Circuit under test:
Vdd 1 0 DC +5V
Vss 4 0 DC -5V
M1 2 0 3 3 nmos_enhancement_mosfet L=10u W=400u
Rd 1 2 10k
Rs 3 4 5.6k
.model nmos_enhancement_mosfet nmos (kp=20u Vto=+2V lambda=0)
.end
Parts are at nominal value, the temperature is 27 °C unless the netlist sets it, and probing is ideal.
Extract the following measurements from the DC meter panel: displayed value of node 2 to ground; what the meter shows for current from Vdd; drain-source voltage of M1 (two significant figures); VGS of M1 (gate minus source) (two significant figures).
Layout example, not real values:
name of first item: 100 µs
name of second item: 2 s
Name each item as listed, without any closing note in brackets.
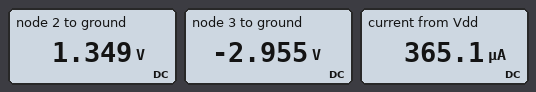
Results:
displayed value of node 2 to ground: 1.349 V
what the meter shows for current from Vdd: 365.1 µA
drain-source voltage of M1: 4.3 V
VGS of M1 (gate minus source): 3.0 V
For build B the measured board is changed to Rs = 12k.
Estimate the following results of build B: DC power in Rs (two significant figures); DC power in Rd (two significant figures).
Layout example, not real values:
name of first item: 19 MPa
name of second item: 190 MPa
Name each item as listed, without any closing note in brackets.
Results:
DC power in Rs: 440 µW
DC power in Rd: 370 µW
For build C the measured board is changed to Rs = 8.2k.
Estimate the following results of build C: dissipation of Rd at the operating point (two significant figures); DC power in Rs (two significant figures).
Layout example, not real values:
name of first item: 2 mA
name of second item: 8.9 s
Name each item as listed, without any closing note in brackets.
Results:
dissipation of Rd at the operating point: 710 µW
DC power in Rs: 580 µW
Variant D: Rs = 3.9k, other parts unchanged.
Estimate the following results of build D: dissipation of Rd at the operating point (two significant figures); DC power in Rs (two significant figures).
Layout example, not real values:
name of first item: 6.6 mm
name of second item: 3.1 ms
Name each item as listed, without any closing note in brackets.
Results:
dissipation of Rd at the operating point: 2.4 mW
DC power in Rs: 920 µW
